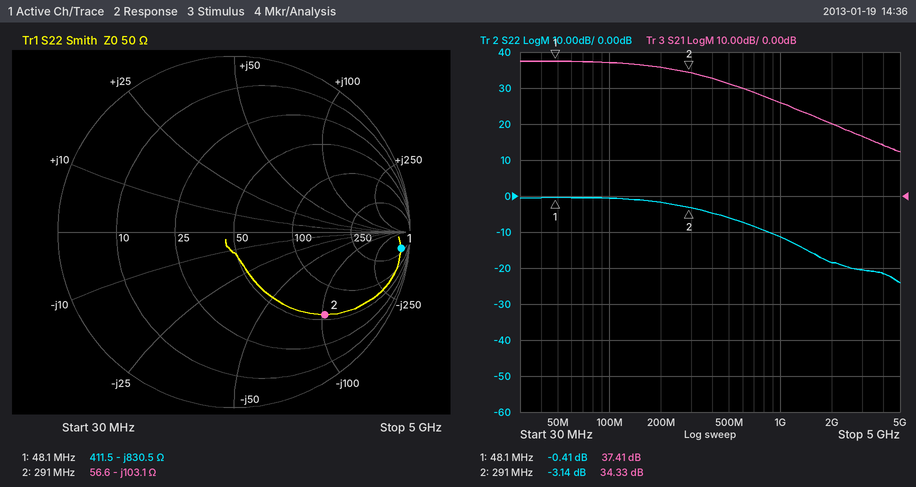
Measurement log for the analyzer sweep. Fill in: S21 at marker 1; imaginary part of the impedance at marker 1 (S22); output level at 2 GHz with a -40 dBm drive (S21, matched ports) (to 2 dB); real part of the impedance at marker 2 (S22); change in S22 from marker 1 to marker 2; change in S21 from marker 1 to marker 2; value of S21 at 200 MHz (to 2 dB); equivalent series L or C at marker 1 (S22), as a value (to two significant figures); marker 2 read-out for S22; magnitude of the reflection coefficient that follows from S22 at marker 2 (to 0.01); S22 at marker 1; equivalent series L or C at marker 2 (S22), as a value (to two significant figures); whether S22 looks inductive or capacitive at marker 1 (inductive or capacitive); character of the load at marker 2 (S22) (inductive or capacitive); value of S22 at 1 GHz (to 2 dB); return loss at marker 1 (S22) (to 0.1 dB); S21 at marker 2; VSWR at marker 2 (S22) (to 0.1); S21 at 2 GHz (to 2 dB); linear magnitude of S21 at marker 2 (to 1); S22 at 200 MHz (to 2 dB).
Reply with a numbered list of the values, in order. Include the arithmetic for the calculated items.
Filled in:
1. 37.41 dB
2. -830.5 Ω
3. -40 dBm + (20 dB) = -20 dBm
4. 56.6 Ω
5. -3.14 − (-0.41) = -2.73 dB
6. 34.33 − (37.41) = -3.08 dB
7. 36 dB
8. C = 1/(2π × 48.1 MHz × 830.5 Ω) ≈ 4.0 pF
9. -3.14 dB
10. 10^(-3.14/20) ≈ 0.70
11. -0.41 dB
12. C = 1/(2π × 291 MHz × 103.1 Ω) ≈ 5.3 pF
13. capacitive
14. capacitive
15. -12 dB
16. 0.4 dB
17. 34.33 dB
18. 5.6
19. 20 dB
20. 10^(34.33/20) ≈ 52
21. -2 dB
